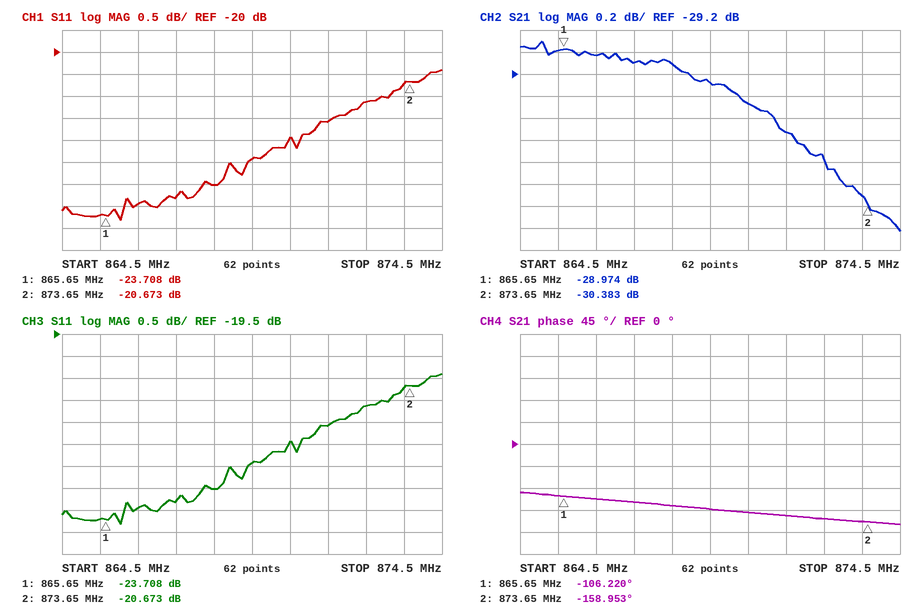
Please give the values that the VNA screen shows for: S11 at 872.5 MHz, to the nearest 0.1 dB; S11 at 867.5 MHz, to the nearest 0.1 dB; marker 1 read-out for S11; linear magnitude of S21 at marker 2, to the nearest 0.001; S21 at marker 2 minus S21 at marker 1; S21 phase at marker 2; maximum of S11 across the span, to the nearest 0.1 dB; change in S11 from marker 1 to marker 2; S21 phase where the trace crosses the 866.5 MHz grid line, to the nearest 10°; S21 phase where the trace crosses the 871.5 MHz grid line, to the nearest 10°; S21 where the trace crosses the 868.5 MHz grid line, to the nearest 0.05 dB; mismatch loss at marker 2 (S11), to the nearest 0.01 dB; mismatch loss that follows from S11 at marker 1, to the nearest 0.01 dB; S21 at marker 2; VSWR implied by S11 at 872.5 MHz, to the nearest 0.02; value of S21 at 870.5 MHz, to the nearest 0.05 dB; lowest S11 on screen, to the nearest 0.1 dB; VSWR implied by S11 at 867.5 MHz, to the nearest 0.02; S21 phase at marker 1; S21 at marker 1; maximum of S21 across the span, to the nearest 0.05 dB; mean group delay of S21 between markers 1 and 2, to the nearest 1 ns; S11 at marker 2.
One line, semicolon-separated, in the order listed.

-21.1 dB; -23.3 dB; -23.708 dB; 0.030; -1.409 dB; -158.953°; -20.4 dB; 3.035 dB; -110°; -150°; -29.10 dB; 0.04 dB; 0.02 dB; -30.383 dB; 1.20; -29.45 dB; -23.8 dB; 1.14; -106.220°; -28.974 dB; -28.90 dB; 18 ns; -20.673 dB
